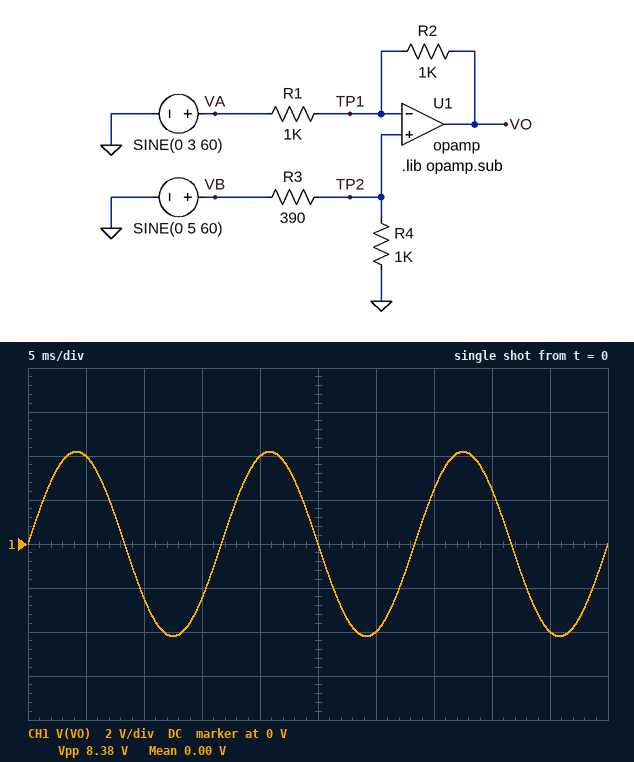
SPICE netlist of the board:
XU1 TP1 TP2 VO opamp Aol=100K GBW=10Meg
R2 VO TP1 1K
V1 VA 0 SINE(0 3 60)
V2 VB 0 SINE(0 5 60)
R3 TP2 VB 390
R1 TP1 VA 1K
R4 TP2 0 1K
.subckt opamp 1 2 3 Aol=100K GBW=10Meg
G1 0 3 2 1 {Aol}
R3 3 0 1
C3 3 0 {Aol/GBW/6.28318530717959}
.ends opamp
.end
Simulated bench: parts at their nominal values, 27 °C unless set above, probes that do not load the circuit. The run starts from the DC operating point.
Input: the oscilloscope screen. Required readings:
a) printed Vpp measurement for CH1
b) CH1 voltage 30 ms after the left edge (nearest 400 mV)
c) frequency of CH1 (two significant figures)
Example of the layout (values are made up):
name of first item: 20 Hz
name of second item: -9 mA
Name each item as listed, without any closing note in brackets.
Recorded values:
printed Vpp measurement for CH1: 8.38 V
CH1 voltage 30 ms after the left edge: -4.0 V
frequency of CH1: 60 Hz
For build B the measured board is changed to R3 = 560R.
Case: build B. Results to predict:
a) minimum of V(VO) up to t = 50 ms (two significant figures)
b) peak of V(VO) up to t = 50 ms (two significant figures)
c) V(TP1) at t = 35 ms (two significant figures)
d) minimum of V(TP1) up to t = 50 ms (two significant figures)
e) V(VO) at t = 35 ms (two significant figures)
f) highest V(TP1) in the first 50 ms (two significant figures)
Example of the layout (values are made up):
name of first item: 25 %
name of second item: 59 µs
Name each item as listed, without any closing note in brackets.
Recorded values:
minimum of V(VO) up to t = 50 ms: -3.4 V
peak of V(VO) up to t = 50 ms: 3.4 V
V(TP1) at t = 35 ms: 1.9 V
minimum of V(TP1) up to t = 50 ms: -3.2 V
V(VO) at t = 35 ms: 2.0 V
highest V(TP1) in the first 50 ms: 3.2 V
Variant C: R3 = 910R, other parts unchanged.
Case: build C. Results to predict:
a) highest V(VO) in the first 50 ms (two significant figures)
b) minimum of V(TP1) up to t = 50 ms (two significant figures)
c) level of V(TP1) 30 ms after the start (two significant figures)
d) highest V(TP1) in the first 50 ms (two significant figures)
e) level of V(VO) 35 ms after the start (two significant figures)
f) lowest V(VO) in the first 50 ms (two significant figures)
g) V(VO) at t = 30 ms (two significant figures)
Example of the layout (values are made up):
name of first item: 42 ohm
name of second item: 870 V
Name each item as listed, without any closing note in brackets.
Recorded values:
highest V(VO) in the first 50 ms: 2.2 V
minimum of V(TP1) up to t = 50 ms: -2.6 V
level of V(TP1) 30 ms after the start: -2.5 V
highest V(TP1) in the first 50 ms: 2.6 V
level of V(VO) 35 ms after the start: 1.3 V
lowest V(VO) in the first 50 ms: -2.2 V
V(VO) at t = 30 ms: -2.1 V
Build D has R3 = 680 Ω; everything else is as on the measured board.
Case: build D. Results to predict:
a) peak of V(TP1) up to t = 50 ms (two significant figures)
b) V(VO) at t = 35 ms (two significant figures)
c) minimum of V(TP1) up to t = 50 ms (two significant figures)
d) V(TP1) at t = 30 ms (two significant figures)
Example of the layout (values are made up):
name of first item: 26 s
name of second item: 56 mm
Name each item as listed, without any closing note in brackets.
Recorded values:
peak of V(TP1) up to t = 50 ms: 3.0 V
V(VO) at t = 35 ms: 1.7 V
minimum of V(TP1) up to t = 50 ms: -3.0 V
V(TP1) at t = 30 ms: -2.8 V
